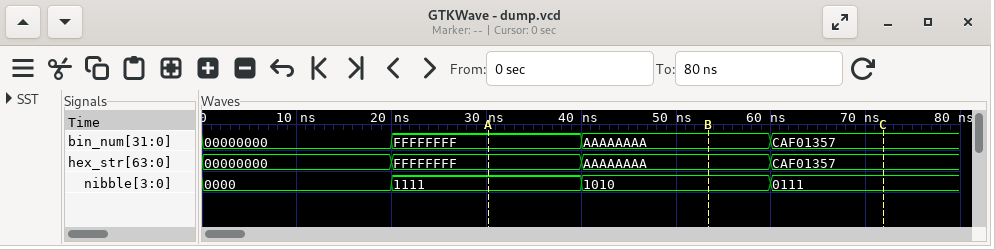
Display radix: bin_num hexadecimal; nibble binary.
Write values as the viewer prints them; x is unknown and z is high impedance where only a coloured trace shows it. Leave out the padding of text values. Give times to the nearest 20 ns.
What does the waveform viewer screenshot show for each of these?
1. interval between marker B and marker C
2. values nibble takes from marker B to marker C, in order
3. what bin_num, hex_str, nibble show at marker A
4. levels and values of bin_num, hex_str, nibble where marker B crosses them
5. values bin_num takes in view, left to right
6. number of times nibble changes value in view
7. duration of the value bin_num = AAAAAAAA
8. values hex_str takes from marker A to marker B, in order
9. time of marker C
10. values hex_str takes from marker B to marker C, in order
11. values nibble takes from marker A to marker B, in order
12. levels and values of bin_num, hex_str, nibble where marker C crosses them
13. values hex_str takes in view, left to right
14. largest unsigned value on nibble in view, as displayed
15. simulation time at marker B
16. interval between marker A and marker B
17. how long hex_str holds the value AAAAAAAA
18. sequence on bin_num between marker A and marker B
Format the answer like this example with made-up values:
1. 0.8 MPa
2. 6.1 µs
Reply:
1. 20 ns
2. 1010, 0111
3. bin_num=FFFFFFFF, hex_str=FFFFFFFF, nibble=1111
4. bin_num=AAAAAAAA, hex_str=AAAAAAAA, nibble=1010
5. 00000000, FFFFFFFF, AAAAAAAA, CAF01357
6. 3
7. 20 ns
8. FFFFFFFF, AAAAAAAA
9. 80 ns
10. AAAAAAAA, CAF01357
11. 1111, 1010
12. bin_num=CAF01357, hex_str=CAF01357, nibble=0111
13. 00000000, FFFFFFFF, AAAAAAAA, CAF01357
14. 1111
15. 60 ns
16. 20 ns
17. 20 ns
18. FFFFFFFF, AAAAAAAA
